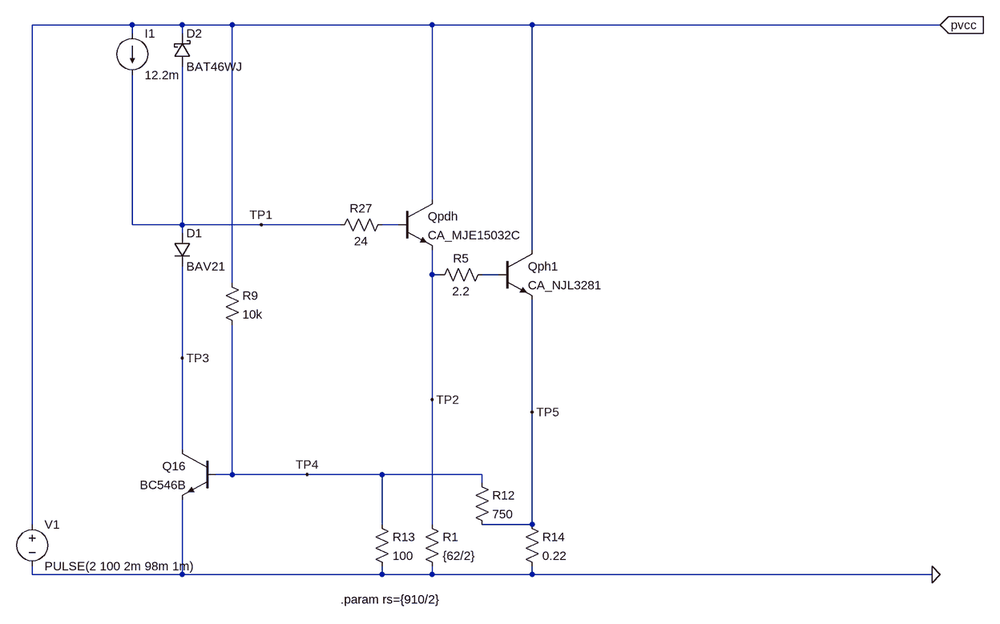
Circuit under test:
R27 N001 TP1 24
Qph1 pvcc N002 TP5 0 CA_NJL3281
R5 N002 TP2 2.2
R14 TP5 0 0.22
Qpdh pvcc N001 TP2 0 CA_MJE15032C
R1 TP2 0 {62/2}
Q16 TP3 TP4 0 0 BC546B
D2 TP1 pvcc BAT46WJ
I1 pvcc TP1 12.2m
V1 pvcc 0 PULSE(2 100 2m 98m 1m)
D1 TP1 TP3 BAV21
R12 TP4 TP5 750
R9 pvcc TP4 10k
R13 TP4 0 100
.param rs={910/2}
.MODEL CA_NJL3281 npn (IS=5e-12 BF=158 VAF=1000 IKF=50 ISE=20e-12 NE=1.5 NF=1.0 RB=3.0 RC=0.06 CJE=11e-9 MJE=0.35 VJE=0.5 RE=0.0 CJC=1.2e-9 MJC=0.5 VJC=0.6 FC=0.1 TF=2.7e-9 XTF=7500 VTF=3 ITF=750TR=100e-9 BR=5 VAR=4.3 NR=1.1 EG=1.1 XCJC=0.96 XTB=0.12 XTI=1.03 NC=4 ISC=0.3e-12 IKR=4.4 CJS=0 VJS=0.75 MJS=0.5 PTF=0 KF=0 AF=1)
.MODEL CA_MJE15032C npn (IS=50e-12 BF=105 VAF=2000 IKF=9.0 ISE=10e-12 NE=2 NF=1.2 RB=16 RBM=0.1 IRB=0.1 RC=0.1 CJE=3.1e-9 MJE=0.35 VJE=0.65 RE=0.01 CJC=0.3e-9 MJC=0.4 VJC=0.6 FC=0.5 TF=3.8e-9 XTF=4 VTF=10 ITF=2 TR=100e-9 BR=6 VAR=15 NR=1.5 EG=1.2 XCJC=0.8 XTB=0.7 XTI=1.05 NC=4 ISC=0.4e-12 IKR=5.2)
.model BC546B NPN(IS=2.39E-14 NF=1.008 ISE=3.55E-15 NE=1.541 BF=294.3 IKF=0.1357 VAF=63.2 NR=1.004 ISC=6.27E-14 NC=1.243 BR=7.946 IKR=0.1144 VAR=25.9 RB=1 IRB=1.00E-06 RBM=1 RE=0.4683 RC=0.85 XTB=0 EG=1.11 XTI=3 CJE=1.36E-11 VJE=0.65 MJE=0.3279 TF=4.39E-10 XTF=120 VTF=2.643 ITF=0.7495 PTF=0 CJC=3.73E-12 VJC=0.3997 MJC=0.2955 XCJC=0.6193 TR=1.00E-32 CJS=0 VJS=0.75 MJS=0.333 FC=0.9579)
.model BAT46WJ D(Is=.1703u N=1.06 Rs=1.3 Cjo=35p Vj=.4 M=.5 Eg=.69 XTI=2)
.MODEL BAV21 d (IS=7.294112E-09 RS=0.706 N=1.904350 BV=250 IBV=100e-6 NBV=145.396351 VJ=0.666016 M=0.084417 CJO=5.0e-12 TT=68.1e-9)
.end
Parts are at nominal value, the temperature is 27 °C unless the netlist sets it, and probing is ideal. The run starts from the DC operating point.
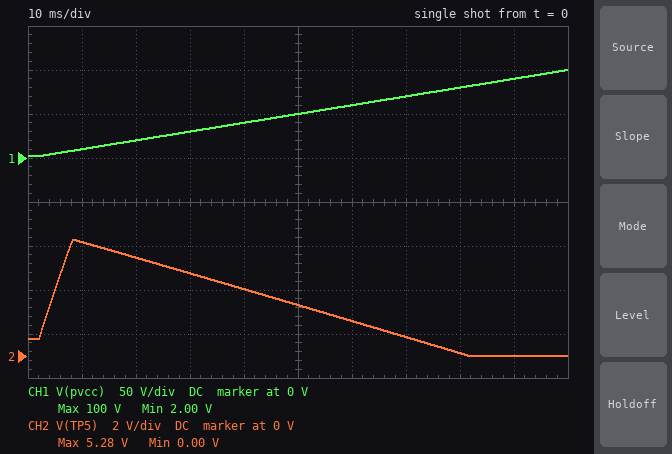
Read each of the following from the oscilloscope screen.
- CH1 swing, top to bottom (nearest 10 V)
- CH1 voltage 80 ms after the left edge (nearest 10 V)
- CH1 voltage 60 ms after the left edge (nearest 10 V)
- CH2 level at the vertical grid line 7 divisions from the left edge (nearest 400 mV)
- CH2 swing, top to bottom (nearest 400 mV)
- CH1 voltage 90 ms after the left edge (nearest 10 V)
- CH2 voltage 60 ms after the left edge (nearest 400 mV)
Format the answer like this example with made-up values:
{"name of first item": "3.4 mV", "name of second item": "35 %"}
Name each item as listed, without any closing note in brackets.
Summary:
{"CH1 swing, top to bottom": "100 V", "CH1 voltage 80 ms after the left edge": "80 V", "CH1 voltage 60 ms after the left edge": "60 V", "CH2 level at the vertical grid line 7 divisions from the left edge": "800 mV", "CH2 swing, top to bottom": "5.2 V", "CH1 voltage 90 ms after the left edge": "90 V", "CH2 voltage 60 ms after the left edge": "1.6 V"}
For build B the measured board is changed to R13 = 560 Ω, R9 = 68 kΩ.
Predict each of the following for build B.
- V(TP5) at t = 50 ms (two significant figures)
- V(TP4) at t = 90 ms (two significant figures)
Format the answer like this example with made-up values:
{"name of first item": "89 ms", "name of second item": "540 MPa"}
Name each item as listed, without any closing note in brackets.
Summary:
{"V(TP5) at t = 50 ms": "1.1 V", "V(TP4) at t = 90 ms": "710 mV"}
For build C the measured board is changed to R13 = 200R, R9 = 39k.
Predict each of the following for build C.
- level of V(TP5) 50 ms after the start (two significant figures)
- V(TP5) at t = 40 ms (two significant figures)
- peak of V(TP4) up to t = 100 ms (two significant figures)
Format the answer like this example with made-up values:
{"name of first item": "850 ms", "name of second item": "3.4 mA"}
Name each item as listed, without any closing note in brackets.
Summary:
{"level of V(TP5) 50 ms after the start": "2.4 V", "V(TP5) at t = 40 ms": "2.6 V", "peak of V(TP4) up to t = 100 ms": "710 mV"}
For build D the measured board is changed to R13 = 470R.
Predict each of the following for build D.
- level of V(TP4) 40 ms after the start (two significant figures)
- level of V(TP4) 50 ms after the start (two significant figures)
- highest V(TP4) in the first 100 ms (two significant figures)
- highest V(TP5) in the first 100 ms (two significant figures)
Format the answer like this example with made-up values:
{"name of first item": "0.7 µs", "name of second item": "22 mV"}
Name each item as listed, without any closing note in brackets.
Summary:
{"level of V(TP4) 40 ms after the start": "730 mV", "level of V(TP4) 50 ms after the start": "740 mV", "highest V(TP4) in the first 100 ms": "770 mV", "highest V(TP5) in the first 100 ms": "1.7 V"}
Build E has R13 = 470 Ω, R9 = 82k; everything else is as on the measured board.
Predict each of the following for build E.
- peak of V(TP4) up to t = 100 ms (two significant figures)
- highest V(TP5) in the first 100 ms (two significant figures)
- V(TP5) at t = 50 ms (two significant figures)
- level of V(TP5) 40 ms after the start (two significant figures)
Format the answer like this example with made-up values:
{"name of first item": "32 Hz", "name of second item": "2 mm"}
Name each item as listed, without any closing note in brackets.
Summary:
{"peak of V(TP4) up to t = 100 ms": "710 mV", "highest V(TP5) in the first 100 ms": "1.8 V", "V(TP5) at t = 50 ms": "1.4 V", "level of V(TP5) 40 ms after the start": "1.5 V"}
